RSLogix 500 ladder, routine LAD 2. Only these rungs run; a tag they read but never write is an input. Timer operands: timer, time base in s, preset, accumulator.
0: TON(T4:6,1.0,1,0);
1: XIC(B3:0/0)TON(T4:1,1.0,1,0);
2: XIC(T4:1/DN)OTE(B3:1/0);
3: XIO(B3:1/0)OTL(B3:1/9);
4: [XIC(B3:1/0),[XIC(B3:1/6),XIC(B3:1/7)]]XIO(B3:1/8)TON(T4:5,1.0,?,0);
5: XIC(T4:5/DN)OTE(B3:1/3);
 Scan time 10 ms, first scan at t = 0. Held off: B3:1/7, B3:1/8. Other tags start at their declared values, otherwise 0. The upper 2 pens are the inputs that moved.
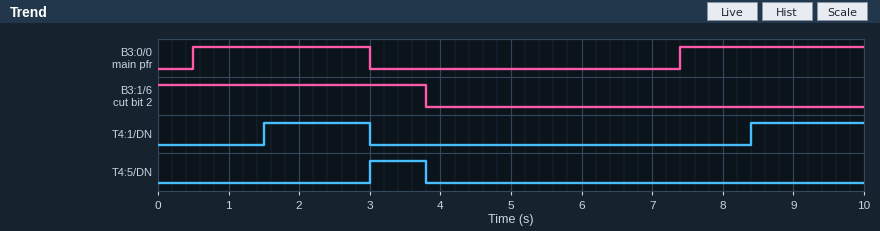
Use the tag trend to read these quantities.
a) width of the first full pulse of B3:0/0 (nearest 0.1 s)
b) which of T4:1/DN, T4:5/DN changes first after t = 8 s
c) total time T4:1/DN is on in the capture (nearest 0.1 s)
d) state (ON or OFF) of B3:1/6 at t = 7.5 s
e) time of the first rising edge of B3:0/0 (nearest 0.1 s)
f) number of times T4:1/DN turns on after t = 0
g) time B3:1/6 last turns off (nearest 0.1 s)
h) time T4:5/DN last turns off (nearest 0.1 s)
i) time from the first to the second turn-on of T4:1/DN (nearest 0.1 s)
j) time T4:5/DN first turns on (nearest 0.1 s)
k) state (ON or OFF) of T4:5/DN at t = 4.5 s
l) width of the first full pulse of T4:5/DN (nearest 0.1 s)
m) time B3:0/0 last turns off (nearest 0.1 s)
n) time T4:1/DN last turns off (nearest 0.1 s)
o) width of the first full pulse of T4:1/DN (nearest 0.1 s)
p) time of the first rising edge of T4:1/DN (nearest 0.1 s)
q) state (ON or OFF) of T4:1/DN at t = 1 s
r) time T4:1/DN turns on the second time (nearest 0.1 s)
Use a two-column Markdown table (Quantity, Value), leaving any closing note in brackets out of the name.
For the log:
| Quantity | Value |
|---|---|
| width of the first full pulse of B3:0/0 | 2.5 s |
| which of T4:1/DN, T4:5/DN changes first after t = 8 s | T4:1/DN |
| total time T4:1/DN is on in the capture | 3.1 s |
| state (ON or OFF) of B3:1/6 at t = 7.5 s | OFF |
| time of the first rising edge of B3:0/0 | 0.5 s |
| number of times T4:1/DN turns on after t = 0 | 2 |
| time B3:1/6 last turns off | 3.8 s |
| time T4:5/DN last turns off | 3.8 s |
| time from the first to the second turn-on of T4:1/DN | 6.9 s |
| time T4:5/DN first turns on | 3.0 s |
| state (ON or OFF) of T4:5/DN at t = 4.5 s | OFF |
| width of the first full pulse of T4:5/DN | 0.8 s |
| time B3:0/0 last turns off | 3.0 s |
| time T4:1/DN last turns off | 3.0 s |
| width of the first full pulse of T4:1/DN | 1.5 s |
| time of the first rising edge of T4:1/DN | 1.5 s |
| state (ON or OFF) of T4:1/DN at t = 1 s | OFF |
| time T4:1/DN turns on the second time | 8.4 s |
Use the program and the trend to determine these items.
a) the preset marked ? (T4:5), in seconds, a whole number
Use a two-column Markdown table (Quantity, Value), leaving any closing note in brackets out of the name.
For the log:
| Quantity | Value |
|---|---|
| the preset marked ? (T4:5), in seconds, a whole number | 3 s |
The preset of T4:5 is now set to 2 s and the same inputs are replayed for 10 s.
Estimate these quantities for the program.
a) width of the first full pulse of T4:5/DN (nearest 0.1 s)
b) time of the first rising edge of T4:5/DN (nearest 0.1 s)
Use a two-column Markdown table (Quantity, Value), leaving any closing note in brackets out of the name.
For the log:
| Quantity | Value |
|---|---|
| width of the first full pulse of T4:5/DN | 1.8 s |
| time of the first rising edge of T4:5/DN | 2.0 s |
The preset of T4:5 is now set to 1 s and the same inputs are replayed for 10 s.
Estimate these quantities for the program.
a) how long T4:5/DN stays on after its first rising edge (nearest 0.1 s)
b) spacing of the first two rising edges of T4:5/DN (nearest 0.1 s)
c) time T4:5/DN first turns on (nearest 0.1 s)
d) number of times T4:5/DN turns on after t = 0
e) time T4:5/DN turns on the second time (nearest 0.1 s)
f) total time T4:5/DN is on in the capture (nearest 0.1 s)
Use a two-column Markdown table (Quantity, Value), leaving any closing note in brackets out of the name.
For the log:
| Quantity | Value |
|---|---|
| how long T4:5/DN stays on after its first rising edge | 2.8 s |
| spacing of the first two rising edges of T4:5/DN | 8.4 s |
| time T4:5/DN first turns on | 1.0 s |
| number of times T4:5/DN turns on after t = 0 | 2 |
| time T4:5/DN turns on the second time | 9.4 s |
| total time T4:5/DN is on in the capture | 3.4 s |
